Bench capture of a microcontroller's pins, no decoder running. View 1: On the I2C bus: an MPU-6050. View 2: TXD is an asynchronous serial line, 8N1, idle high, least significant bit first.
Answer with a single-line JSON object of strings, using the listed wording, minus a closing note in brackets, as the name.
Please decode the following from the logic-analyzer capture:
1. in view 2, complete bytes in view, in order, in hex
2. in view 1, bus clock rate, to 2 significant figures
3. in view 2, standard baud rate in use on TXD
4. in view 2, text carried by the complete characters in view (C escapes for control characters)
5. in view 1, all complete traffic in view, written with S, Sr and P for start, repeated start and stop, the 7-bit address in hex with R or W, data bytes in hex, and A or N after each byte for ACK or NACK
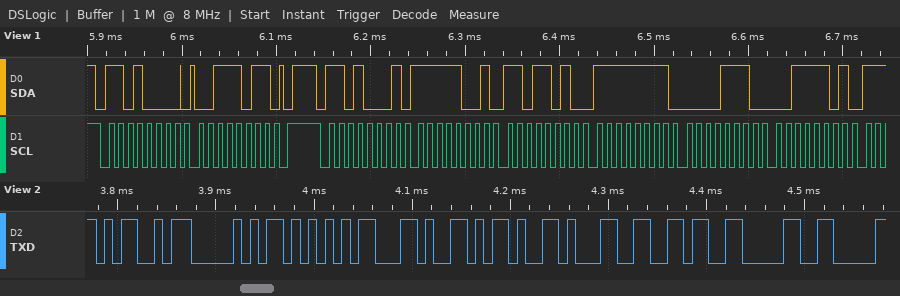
{"in view 2, complete bytes in view, in order, in hex": "4D 50 55 2C 2D 31 36 30", "in view 1, bus clock rate, to 2 significant figures": "100 kHz", "in view 2, standard baud rate in use on TXD": "115200 baud", "in view 2, text carried by the complete characters in view": "\"MPU,-160\"", "in view 1, all complete traffic in view, written with S, Sr and P for start, repeated start and stop, the 7-bit address in hex with R or W, data bytes in hex, and A or N after each byte for ACK or NACK": "S 68W A 3B A P S 68R A F9 A DA A FF A 0E A 3D A"}
